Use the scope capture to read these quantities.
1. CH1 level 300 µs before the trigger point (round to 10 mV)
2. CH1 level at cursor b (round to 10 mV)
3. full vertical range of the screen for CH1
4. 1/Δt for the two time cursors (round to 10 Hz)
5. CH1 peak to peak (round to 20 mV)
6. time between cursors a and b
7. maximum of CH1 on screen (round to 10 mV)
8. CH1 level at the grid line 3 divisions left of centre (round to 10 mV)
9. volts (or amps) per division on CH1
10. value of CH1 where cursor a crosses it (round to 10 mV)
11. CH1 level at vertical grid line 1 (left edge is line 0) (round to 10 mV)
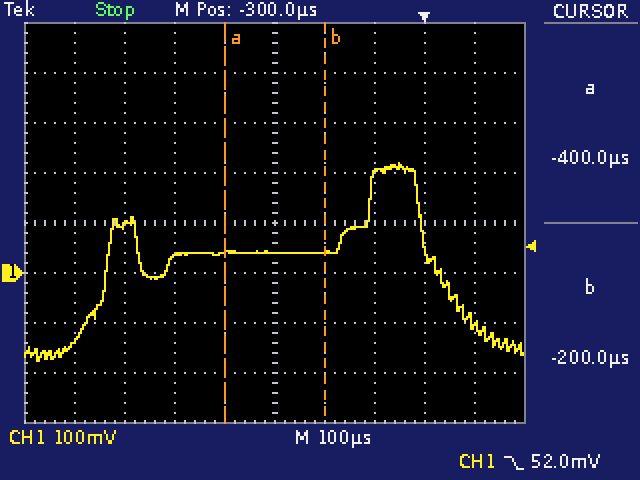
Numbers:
40 mV
40 mV
800 mV
5.00 kHz
400 mV
200 µs
220 mV
100 mV
100 mV
40 mV
-140 mV
